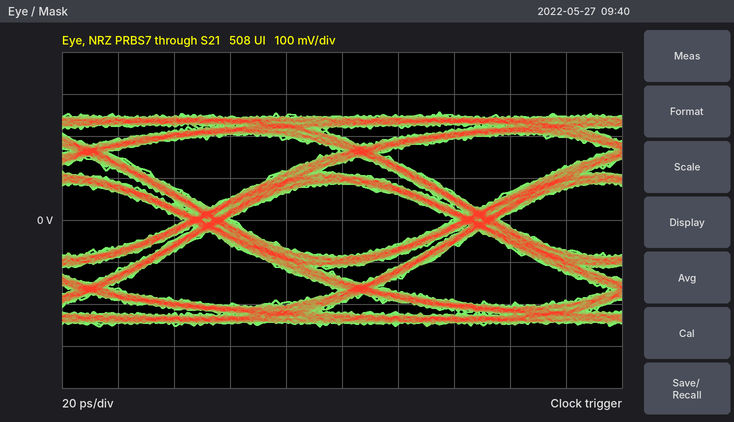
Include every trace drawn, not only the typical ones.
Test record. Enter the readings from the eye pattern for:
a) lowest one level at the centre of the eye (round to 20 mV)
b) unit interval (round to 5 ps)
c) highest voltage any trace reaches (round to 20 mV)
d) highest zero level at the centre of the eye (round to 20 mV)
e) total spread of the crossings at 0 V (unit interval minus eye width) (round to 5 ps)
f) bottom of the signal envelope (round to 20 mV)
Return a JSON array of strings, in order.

["80 mV", "95 ps", "260 mV", "-80 mV", "20 ps", "-260 mV"]
